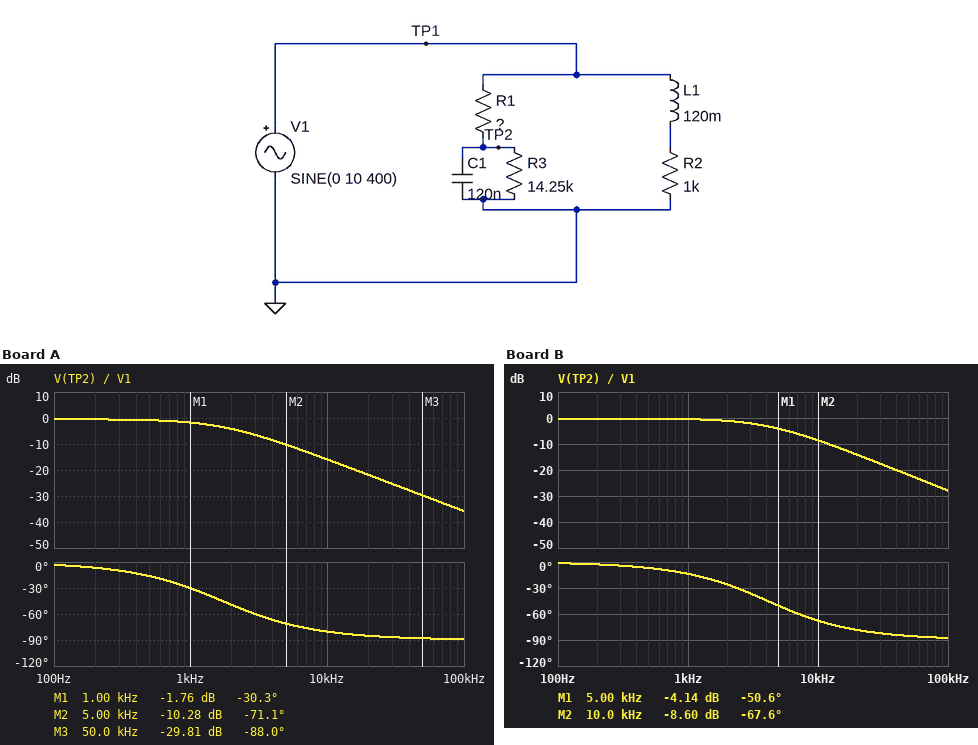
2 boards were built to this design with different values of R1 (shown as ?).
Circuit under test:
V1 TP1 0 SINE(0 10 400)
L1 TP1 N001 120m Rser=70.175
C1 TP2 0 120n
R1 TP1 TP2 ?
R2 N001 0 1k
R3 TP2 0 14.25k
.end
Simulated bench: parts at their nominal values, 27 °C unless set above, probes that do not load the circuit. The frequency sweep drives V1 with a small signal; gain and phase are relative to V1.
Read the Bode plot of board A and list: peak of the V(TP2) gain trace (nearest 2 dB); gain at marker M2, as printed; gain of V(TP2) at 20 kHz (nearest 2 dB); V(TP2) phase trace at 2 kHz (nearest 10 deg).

0 dB
-10.28 dB
-22 dB
-50 deg
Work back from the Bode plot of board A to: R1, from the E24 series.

820 Ω
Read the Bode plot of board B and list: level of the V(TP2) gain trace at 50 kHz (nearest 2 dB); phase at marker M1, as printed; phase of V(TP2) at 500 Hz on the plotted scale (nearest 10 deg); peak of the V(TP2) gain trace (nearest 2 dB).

-22 dB
-50.6 deg
-10 deg
0 dB
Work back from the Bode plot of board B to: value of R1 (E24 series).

330 Ω
